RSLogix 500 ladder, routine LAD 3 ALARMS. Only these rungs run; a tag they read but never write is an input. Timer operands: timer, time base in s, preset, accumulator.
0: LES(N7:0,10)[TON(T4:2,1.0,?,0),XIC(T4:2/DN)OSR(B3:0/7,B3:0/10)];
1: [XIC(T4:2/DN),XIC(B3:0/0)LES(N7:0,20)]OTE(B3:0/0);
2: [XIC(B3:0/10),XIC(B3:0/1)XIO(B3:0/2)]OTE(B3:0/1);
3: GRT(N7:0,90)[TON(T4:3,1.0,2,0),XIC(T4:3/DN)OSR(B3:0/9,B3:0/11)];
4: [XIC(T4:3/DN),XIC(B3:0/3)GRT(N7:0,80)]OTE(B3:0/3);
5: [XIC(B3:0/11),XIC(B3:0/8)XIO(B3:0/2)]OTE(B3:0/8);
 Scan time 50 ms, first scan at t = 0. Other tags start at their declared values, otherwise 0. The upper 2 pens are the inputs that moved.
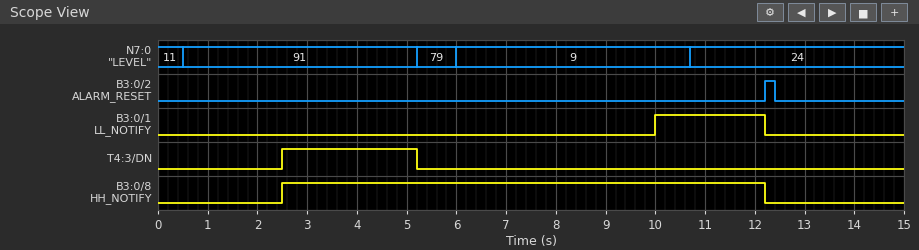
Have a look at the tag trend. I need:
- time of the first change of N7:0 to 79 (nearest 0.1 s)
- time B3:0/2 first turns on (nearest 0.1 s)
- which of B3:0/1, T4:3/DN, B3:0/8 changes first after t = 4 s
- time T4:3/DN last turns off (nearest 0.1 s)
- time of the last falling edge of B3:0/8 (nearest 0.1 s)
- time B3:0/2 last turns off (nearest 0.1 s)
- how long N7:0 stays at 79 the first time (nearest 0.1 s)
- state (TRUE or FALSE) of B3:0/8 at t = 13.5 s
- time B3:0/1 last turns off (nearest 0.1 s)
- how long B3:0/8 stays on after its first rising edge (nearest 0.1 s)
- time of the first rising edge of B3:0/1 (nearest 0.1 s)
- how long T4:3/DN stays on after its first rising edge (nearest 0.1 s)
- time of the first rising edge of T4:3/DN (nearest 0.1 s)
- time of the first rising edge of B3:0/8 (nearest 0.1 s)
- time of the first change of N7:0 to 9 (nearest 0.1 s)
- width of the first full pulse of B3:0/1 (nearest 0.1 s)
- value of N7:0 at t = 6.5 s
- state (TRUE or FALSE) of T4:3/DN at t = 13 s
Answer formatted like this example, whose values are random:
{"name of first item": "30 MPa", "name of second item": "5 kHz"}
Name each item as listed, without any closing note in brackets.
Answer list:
{"time of the first change of N7:0 to 79": "5.2 s", "time B3:0/2 first turns on": "12.2 s", "which of B3:0/1, T4:3/DN, B3:0/8 changes first after t = 4 s": "T4:3/DN", "time T4:3/DN last turns off": "5.2 s", "time of the last falling edge of B3:0/8": "12.2 s", "time B3:0/2 last turns off": "12.4 s", "how long N7:0 stays at 79 the first time": "0.8 s", "state (TRUE or FALSE) of B3:0/8 at t = 13.5 s": "FALSE", "time B3:0/1 last turns off": "12.2 s", "how long B3:0/8 stays on after its first rising edge": "9.7 s", "time of the first rising edge of B3:0/1": "10.0 s", "how long T4:3/DN stays on after its first rising edge": "2.7 s", "time of the first rising edge of T4:3/DN": "2.5 s", "time of the first rising edge of B3:0/8": "2.5 s", "time of the first change of N7:0 to 9": "6.0 s", "width of the first full pulse of B3:0/1": "2.2 s", "value of N7:0 at t = 6.5 s": "9", "state (TRUE or FALSE) of T4:3/DN at t = 13 s": "FALSE"}
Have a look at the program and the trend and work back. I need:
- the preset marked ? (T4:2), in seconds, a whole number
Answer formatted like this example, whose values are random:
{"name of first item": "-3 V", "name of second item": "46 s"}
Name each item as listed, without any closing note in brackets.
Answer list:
{"the preset marked ? (T4:2), in seconds, a whole number": "4 s"}
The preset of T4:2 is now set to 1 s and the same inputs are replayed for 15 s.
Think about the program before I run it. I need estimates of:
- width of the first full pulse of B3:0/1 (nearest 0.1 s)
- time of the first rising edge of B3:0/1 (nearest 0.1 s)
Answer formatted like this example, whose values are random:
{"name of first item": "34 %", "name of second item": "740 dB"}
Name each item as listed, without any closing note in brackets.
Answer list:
{"width of the first full pulse of B3:0/1": "5.2 s", "time of the first rising edge of B3:0/1": "7.0 s"}
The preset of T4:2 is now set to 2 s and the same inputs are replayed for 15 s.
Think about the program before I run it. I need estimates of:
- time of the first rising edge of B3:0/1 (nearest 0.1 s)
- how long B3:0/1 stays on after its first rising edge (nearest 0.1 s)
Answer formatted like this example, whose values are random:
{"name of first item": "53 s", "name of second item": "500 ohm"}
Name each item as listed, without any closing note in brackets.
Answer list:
{"time of the first rising edge of B3:0/1": "8.0 s", "how long B3:0/1 stays on after its first rising edge": "4.2 s"}
